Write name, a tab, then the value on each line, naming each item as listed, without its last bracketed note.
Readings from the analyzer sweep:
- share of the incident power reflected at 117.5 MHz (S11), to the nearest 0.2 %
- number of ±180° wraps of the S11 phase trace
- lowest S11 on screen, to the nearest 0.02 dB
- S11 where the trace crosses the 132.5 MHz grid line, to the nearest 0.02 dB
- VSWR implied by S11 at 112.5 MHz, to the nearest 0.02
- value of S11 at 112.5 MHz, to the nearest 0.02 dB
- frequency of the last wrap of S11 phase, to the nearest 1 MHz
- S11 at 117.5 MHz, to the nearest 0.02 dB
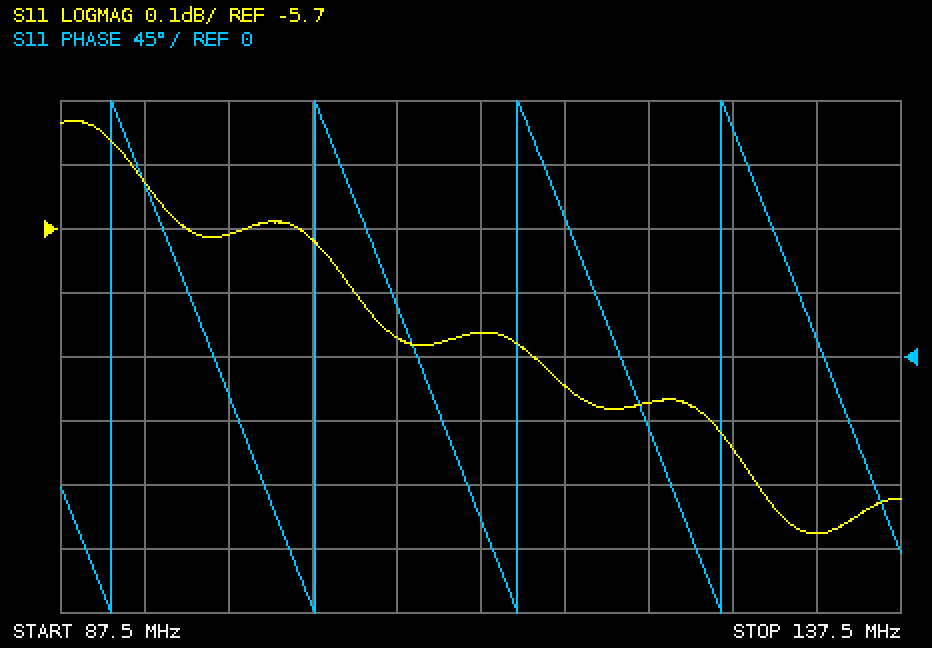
share of the incident power reflected at 117.5 MHz (S11), to the nearest 0.2 %	25.4 %
number of ±180° wraps of the S11 phase trace	4
lowest S11 on screen, to the nearest 0.02 dB	-6.18 dB
S11 where the trace crosses the 132.5 MHz grid line, to the nearest 0.02 dB	-6.18 dB
VSWR implied by S11 at 112.5 MHz, to the nearest 0.02	3.08
value of S11 at 112.5 MHz, to the nearest 0.02 dB	-5.86 dB
frequency of the last wrap of S11 phase, to the nearest 1 MHz	127 MHz
S11 at 117.5 MHz, to the nearest 0.02 dB	-5.94 dB
